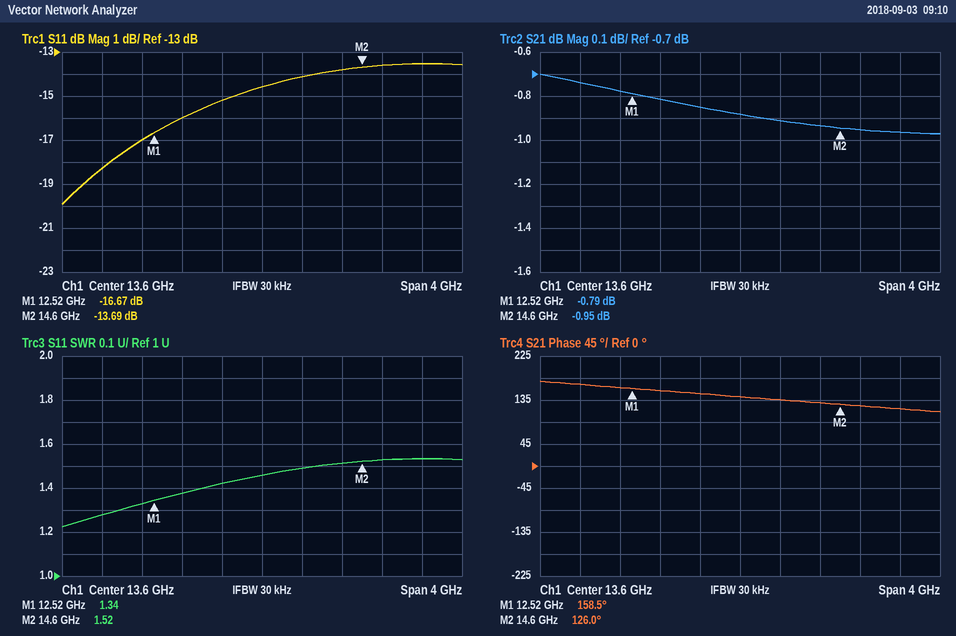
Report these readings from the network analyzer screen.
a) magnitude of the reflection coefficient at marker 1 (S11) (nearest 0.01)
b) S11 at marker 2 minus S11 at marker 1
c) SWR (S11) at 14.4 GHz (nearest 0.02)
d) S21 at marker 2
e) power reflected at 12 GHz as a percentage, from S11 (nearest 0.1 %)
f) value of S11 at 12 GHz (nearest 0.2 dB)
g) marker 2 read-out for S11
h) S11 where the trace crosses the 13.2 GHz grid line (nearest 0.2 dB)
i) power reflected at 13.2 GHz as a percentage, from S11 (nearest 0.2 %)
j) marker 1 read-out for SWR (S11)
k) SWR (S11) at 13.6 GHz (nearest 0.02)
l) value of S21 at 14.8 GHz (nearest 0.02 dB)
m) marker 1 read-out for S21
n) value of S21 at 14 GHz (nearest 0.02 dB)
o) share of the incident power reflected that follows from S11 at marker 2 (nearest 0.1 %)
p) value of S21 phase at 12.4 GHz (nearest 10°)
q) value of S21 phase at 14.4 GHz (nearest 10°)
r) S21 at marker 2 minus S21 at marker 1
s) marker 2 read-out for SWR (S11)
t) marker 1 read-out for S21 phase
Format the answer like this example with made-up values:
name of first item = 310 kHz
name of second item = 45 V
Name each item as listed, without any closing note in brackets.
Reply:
magnitude of the reflection coefficient at marker 1 (S11) = 0.15
S11 at marker 2 minus S11 at marker 1 = 2.98 dB
SWR (S11) at 14.4 GHz = 1.52
S21 at marker 2 = -0.95 dB
power reflected at 12 GHz as a percentage, from S11 = 1.5 %
value of S11 at 12 GHz = -18.2 dB
marker 2 read-out for S11 = -13.69 dB
S11 where the trace crosses the 13.2 GHz grid line = -15.2 dB
power reflected at 13.2 GHz as a percentage, from S11 = 3.0 %
marker 1 read-out for SWR = 1.34
SWR (S11) at 13.6 GHz = 1.46
value of S21 at 14.8 GHz = -0.96 dB
marker 1 read-out for S21 = -0.79 dB
value of S21 at 14 GHz = -0.92 dB
share of the incident power reflected that follows from S11 at marker 2 = 4.3 %
value of S21 phase at 12.4 GHz = 160°
value of S21 phase at 14.4 GHz = 130°
S21 at marker 2 minus S21 at marker 1 = -0.16 dB
marker 2 read-out for SWR = 1.52
marker 1 read-out for S21 phase = 158.5°
